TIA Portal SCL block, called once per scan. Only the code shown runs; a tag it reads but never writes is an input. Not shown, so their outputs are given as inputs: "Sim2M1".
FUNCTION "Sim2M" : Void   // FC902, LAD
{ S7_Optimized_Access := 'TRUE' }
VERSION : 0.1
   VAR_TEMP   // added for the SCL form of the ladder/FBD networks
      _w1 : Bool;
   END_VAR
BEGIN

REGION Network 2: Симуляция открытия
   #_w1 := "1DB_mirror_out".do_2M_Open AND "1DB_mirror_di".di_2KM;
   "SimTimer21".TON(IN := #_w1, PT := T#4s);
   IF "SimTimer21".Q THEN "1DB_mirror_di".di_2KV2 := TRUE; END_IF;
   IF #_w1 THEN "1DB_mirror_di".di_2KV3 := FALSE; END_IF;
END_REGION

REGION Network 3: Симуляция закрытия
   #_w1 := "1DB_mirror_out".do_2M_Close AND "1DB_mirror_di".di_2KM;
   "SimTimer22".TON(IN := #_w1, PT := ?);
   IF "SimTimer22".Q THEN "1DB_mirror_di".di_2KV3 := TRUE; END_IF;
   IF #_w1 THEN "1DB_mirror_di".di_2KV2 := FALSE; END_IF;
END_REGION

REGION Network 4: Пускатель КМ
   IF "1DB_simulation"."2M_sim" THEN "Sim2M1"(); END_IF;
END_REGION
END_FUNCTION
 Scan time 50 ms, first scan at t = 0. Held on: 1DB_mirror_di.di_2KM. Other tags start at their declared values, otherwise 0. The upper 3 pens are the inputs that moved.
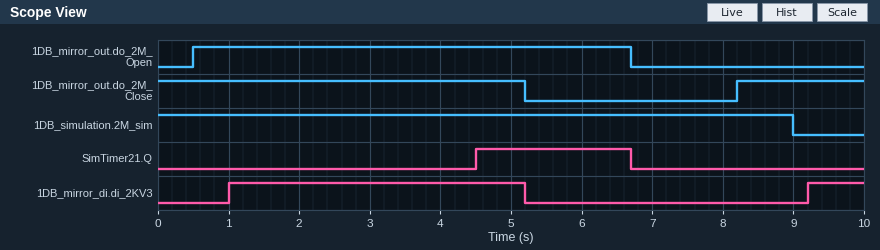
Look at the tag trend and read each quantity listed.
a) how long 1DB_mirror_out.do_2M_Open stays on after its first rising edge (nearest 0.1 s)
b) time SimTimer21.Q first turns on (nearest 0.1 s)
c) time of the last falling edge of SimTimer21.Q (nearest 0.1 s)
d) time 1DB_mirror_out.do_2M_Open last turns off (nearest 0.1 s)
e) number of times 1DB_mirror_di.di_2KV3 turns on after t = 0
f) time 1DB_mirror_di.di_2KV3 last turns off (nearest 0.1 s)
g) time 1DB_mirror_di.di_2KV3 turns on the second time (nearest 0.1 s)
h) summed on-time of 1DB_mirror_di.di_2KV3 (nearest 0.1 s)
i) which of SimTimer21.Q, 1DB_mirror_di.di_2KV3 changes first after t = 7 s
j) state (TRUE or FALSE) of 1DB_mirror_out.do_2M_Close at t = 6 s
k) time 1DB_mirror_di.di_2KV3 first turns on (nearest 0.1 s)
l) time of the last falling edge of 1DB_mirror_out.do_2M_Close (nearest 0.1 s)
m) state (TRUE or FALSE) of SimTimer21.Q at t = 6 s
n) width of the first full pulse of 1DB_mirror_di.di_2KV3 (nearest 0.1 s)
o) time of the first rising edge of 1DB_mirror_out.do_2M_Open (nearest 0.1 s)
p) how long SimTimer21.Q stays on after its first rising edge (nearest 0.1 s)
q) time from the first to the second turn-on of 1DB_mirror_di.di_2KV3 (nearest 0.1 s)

6.2 s
4.5 s
6.7 s
6.7 s
2
5.2 s
9.2 s
5.0 s
1DB_mirror_di.di_2KV3
FALSE
1.0 s
5.2 s
TRUE
4.2 s
0.5 s
2.2 s
8.2 s
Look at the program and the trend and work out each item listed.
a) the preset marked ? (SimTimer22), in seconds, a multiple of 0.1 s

1.0 s
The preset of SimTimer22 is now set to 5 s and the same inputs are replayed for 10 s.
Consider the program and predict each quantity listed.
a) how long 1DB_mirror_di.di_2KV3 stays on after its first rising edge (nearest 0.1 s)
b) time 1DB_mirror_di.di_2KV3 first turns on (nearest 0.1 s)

0.2 s
5.0 s
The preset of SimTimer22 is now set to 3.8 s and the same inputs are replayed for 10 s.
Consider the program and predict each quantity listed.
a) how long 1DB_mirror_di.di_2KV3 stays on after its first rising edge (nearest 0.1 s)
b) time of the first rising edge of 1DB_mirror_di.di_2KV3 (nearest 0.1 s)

1.4 s
3.8 s
